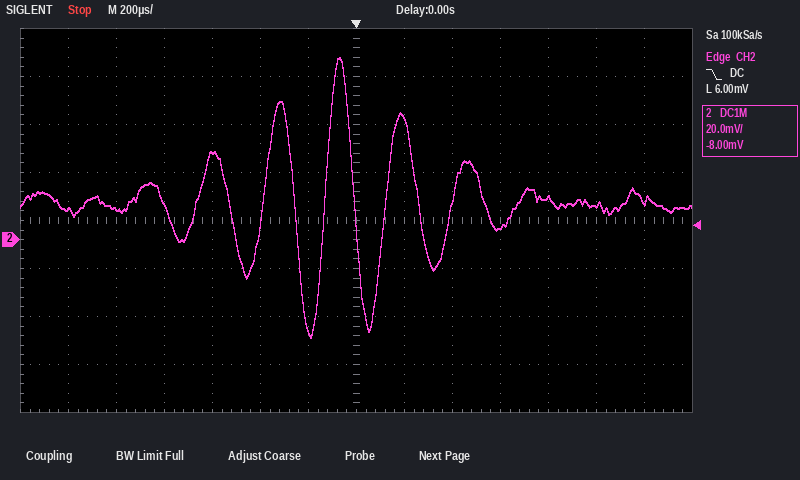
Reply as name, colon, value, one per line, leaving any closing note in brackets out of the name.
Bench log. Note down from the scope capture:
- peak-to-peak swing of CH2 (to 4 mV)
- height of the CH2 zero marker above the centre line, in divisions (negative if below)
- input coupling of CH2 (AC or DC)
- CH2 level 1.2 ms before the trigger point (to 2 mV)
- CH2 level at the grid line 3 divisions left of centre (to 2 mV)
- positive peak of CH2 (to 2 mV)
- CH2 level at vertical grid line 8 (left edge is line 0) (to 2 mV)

peak-to-peak swing of CH2: 116 mV
height of the CH2 zero marker above the centre line, in divisions: -0.4 div
input coupling of CH2: DC
CH2 level 1.2 ms before the trigger point: 12 mV
CH2 level at the grid line 3 divisions left of centre: 36 mV
positive peak of CH2: 76 mV
CH2 level at vertical grid line 8 (left edge is line 0): 50 mV
